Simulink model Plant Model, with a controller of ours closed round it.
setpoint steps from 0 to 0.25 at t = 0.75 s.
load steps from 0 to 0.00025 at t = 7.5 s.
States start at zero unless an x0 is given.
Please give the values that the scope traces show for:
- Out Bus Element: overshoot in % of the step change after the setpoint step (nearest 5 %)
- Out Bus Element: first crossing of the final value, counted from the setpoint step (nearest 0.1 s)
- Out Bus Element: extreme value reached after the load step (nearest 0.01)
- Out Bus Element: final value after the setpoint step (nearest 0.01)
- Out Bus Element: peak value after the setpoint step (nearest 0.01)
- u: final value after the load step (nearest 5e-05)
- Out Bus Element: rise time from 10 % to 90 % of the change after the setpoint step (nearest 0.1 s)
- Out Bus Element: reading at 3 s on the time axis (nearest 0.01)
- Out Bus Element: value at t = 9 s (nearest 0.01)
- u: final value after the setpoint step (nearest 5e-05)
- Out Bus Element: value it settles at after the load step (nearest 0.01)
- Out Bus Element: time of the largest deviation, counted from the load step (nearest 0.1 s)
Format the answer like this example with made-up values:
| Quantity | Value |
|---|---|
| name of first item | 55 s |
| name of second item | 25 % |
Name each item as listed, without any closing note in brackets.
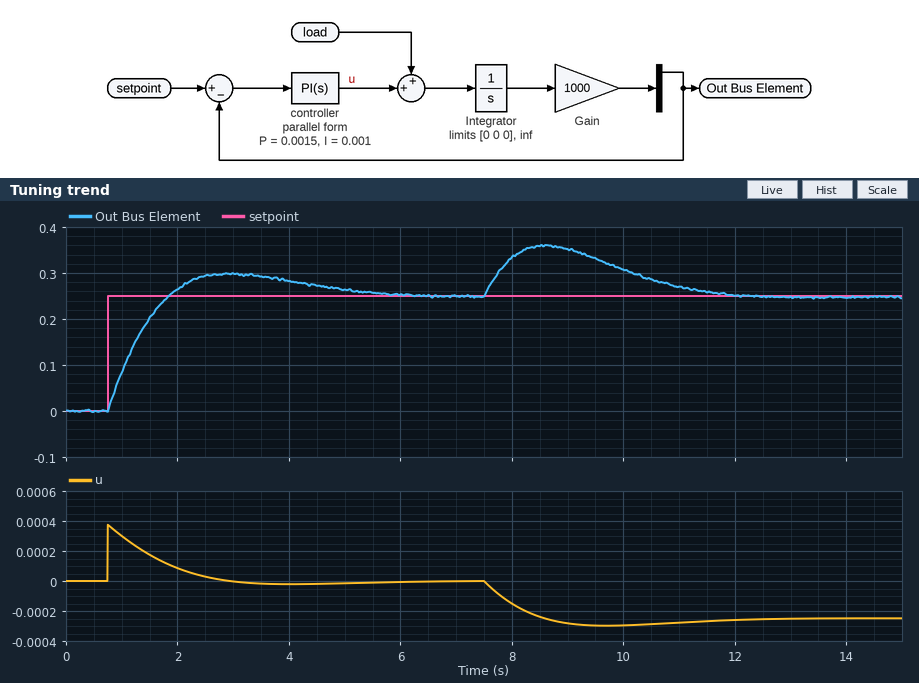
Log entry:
| Quantity | Value |
|---|---|
| Out Bus Element: overshoot in % of the step change after the setpoint step | 20 % |
| Out Bus Element: first crossing of the final value, counted from the setpoint step | 1.1 s |
| Out Bus Element: extreme value reached after the load step | 0.36 |
| Out Bus Element: final value after the setpoint step | 0.25 |
| Out Bus Element: peak value after the setpoint step | 0.30 |
| u: final value after the load step | -0.00025 |
| Out Bus Element: rise time from 10 % to 90 % of the change after the setpoint step | 0.8 s |
| Out Bus Element: reading at 3 s on the time axis | 0.30 |
| Out Bus Element: value at t = 9 s | 0.35 |
| u: final value after the setpoint step | 0.00000 |
| Out Bus Element: value it settles at after the load step | 0.25 |
| Out Bus Element: time of the largest deviation, counted from the load step | 1.1 s |
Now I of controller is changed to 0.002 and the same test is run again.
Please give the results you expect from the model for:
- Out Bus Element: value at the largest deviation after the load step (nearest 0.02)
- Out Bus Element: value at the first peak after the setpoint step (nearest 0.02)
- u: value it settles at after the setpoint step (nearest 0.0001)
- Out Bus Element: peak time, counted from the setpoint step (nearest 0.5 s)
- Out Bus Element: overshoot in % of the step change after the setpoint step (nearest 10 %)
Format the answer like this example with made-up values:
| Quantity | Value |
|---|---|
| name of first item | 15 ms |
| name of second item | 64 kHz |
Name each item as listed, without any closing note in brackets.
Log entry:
| Quantity | Value |
|---|---|
| Out Bus Element: value at the largest deviation after the load step | 0.34 |
| Out Bus Element: value at the first peak after the setpoint step | 0.32 |
| u: value it settles at after the setpoint step | 0.0000 |
| Out Bus Element: peak time, counted from the setpoint step | 1.5 s |
| Out Bus Element: overshoot in % of the step change after the setpoint step | 30 % |
